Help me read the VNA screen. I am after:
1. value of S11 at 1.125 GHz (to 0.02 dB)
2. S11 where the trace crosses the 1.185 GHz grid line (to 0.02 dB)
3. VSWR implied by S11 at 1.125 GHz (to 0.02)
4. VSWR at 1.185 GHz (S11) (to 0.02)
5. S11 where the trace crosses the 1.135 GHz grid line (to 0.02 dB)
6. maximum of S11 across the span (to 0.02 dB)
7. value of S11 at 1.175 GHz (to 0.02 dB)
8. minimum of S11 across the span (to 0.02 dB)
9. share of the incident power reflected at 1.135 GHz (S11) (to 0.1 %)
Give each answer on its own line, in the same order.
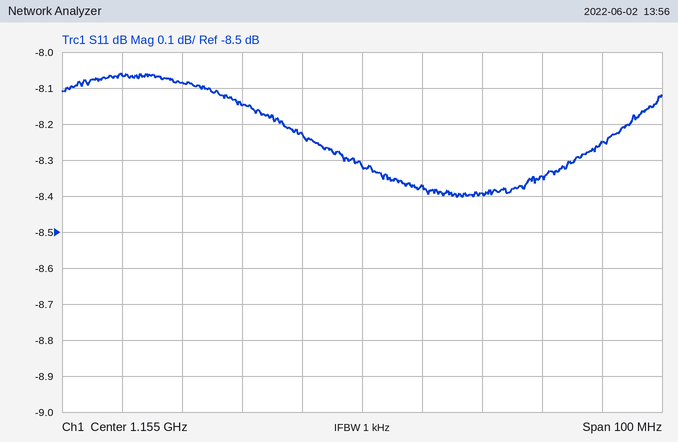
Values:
-8.08 dB
-8.34 dB
2.30
2.24
-8.14 dB
-8.06 dB
-8.40 dB
-8.40 dB
15.3 %
